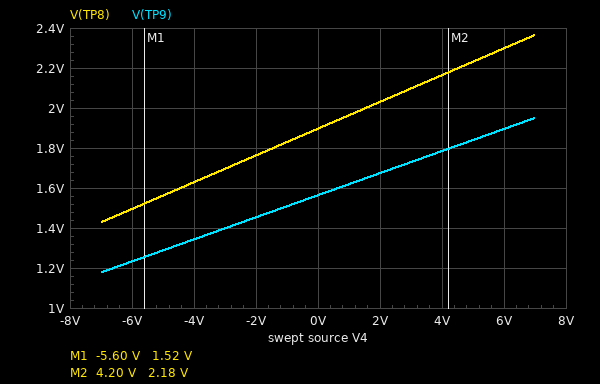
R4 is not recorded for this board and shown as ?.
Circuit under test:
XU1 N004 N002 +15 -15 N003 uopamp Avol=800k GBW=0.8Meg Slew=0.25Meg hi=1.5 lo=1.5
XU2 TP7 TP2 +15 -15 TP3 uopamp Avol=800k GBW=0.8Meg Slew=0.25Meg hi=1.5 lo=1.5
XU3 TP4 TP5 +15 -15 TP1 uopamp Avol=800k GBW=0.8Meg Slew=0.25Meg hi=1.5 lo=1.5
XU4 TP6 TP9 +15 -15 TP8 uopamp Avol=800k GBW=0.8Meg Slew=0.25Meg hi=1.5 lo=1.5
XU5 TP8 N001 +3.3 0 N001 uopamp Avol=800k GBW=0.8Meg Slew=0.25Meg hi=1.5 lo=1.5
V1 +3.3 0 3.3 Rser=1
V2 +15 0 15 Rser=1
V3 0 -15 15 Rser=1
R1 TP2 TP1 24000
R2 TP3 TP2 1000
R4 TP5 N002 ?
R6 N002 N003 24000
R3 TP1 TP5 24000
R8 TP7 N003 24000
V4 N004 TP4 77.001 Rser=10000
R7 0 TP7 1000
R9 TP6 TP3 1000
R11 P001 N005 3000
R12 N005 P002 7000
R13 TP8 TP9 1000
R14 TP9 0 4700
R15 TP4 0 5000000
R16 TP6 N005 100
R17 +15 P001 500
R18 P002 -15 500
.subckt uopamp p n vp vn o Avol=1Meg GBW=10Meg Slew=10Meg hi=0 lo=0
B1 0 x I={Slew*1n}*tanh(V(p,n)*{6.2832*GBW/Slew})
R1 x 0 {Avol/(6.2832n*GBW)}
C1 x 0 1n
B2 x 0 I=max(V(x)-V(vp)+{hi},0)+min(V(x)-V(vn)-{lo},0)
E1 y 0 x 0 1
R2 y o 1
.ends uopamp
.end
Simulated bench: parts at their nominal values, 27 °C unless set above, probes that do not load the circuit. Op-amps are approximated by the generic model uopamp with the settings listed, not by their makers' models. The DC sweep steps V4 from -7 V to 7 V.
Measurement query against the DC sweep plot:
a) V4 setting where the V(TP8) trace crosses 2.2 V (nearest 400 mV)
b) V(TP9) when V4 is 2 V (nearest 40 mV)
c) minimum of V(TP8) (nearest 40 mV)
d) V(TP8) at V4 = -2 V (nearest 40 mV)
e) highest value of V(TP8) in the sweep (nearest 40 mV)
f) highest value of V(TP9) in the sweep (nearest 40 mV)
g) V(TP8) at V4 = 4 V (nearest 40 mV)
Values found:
4.4 V
1.68 V
1.44 V
1.76 V
2.36 V
1.96 V
2.16 V
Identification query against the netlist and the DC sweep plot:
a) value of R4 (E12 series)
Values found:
56 kΩ
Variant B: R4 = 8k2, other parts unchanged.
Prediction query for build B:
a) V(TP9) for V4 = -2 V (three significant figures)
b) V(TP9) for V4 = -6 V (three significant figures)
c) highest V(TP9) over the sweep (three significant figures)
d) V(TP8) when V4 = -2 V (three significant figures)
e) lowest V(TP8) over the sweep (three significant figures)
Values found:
1.16 V
864 mV
2.26 V
1.40 V
1.05 V
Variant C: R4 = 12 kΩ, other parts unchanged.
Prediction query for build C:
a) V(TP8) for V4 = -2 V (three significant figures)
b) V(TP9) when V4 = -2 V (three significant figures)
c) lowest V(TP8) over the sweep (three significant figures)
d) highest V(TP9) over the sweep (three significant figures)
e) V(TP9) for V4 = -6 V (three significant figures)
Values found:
1.54 V
1.27 V
1.09 V
2.23 V
895 mV
